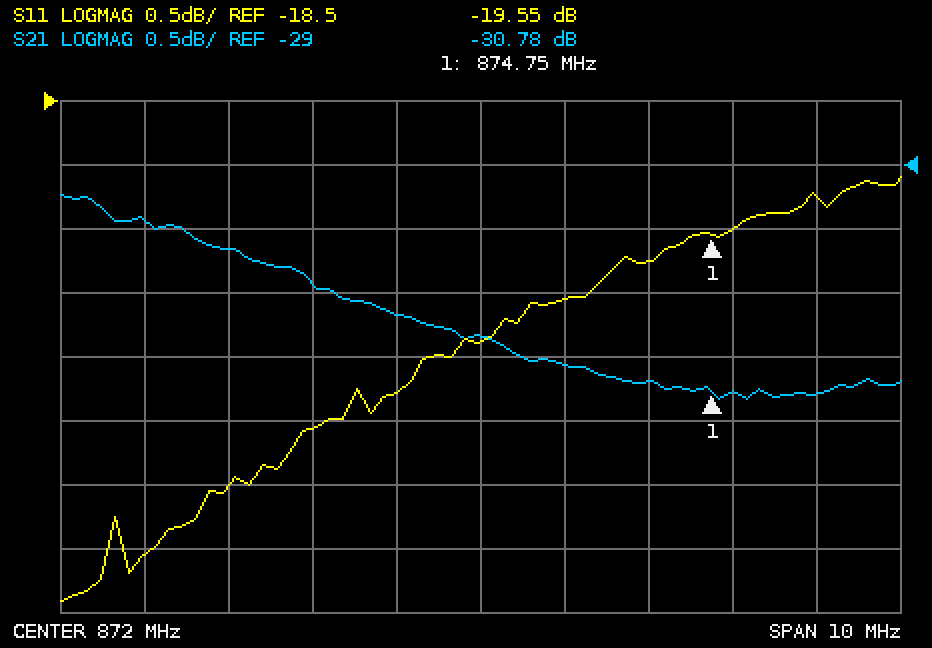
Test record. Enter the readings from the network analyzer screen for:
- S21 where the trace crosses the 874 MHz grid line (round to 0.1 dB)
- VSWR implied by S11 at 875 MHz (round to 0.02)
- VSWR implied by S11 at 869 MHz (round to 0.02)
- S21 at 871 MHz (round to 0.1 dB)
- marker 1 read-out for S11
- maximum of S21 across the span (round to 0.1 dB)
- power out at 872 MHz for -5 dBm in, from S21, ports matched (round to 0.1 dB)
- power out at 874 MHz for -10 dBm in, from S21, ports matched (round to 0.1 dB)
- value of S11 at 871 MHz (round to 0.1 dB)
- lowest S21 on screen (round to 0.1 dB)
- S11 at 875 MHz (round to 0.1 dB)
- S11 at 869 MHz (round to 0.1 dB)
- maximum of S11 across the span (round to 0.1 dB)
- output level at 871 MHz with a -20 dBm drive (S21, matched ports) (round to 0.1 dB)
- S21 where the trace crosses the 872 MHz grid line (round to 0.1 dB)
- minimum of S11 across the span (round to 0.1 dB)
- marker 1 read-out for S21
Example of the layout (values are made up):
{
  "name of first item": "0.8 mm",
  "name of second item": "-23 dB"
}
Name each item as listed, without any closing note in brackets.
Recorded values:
{
  "S21 where the trace crosses the 874 MHz grid line": "-30.7 dB",
  "VSWR implied by S11 at 875 MHz": "1.24",
  "VSWR implied by S11 at 869 MHz": "1.18",
  "S21 at 871 MHz": "-30.2 dB",
  "marker 1 read-out for S11": "-19.55 dB",
  "maximum of S21 across the span": "-29.2 dB",
  "power out at 872 MHz for -5 dBm in, from S21, ports matched": "-35.3 dBm",
  "power out at 874 MHz for -10 dBm in, from S21, ports matched": "-40.7 dBm",
  "value of S11 at 871 MHz": "-20.8 dB",
  "lowest S21 on screen": "-30.8 dB",
  "S11 at 875 MHz": "-19.5 dB",
  "S11 at 869 MHz": "-21.5 dB",
  "maximum of S11 across the span": "-19.1 dB",
  "output level at 871 MHz with a -20 dBm drive (S21, matched ports)": "-50.2 dBm",
  "S21 where the trace crosses the 872 MHz grid line": "-30.3 dB",
  "minimum of S11 across the span": "-22.4 dB",
  "marker 1 read-out for S21": "-30.78 dB"
}
